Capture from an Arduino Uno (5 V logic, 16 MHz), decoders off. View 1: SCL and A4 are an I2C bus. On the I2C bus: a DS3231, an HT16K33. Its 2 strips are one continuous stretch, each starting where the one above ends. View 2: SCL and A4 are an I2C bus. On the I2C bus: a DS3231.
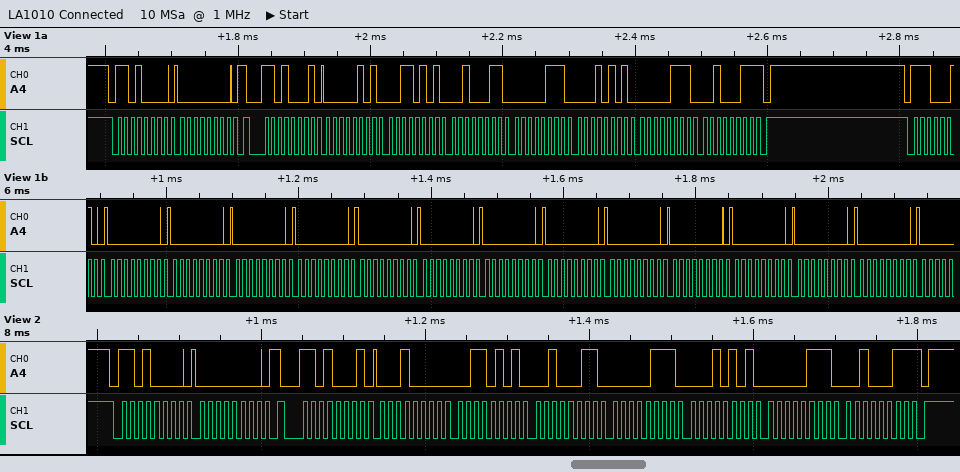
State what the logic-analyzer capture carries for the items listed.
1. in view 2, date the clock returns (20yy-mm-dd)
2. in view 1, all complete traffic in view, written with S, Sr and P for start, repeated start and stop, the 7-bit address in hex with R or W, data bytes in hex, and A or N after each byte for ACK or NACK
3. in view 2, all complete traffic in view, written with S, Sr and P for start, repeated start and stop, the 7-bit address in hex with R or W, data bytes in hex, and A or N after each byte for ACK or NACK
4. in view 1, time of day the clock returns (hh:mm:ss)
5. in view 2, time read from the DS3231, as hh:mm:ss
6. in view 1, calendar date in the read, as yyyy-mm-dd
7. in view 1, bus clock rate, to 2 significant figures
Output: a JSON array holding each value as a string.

["2023-07-15", "S 68W A 00 A Sr 68R A 05 A 35 A 23 A 07 A 15 A 07 A 23 N P S 71W A 00 A 00 A 00 A 00 A 00 A 00 A 00 A 00 A 00 A 00 A 00 A 00 A 00 A", "S 68W A 00 A Sr 68R A 10 A 35 A 23 A 07 A 15 A 07 A 23 N P", "23:35:05", "23:35:10", "2023-07-15", "100 kHz"]
